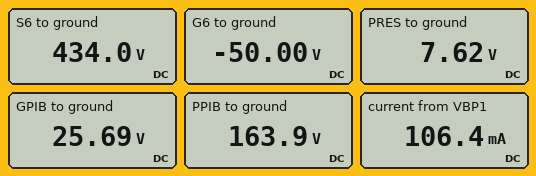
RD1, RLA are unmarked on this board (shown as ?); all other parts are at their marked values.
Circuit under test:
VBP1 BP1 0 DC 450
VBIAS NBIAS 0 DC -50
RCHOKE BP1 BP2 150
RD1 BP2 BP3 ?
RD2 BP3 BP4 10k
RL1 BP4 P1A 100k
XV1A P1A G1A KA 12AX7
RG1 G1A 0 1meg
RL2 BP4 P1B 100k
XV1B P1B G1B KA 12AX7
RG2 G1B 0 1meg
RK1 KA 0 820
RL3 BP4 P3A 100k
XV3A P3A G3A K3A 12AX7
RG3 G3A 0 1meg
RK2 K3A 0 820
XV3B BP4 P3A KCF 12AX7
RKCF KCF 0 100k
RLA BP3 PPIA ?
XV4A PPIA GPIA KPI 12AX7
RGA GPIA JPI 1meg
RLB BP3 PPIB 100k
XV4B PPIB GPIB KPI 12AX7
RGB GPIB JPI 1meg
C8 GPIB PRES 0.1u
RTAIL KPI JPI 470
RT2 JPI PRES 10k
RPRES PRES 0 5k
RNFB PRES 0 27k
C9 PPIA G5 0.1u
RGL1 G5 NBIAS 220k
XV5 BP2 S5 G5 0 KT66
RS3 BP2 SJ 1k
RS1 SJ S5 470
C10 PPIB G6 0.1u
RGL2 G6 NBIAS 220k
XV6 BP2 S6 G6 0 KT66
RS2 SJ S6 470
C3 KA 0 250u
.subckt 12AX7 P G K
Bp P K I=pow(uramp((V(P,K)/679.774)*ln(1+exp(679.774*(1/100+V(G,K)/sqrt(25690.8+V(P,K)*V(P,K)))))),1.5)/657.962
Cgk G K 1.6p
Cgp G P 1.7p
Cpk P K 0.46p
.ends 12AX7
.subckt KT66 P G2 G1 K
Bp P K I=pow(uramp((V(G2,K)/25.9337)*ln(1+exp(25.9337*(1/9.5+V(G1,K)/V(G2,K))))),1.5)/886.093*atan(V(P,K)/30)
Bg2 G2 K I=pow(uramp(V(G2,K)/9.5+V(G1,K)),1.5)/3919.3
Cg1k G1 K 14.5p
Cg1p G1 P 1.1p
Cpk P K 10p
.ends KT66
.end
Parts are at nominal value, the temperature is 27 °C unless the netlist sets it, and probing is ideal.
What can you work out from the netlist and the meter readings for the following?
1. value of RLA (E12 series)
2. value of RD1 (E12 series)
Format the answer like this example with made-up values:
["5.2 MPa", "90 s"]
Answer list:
["220 kΩ", "27 kΩ"]
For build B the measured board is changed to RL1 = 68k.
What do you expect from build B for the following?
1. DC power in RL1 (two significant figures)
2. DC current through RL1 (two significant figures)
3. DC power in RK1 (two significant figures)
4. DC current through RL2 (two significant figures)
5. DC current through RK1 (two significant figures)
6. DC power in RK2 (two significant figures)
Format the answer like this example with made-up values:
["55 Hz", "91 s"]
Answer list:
["58 mW", "930 µA", "2.3 mW", "760 µA", "1.7 mA", "880 µW"]
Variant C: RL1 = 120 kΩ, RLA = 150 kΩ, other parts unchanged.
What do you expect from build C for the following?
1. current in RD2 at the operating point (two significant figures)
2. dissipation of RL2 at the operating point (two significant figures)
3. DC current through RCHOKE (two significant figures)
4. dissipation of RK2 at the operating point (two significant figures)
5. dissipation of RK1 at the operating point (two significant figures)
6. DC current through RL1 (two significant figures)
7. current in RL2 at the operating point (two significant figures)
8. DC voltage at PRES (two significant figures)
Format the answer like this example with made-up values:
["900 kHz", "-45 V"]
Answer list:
["3.9 mA", "67 mW", "110 mA", "890 µW", "2.0 mW", "740 µA", "820 µA", "8.1 V"]
